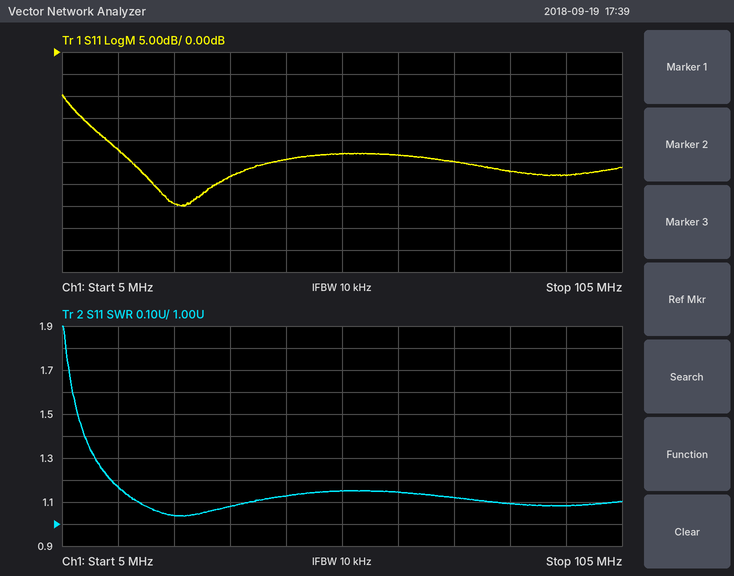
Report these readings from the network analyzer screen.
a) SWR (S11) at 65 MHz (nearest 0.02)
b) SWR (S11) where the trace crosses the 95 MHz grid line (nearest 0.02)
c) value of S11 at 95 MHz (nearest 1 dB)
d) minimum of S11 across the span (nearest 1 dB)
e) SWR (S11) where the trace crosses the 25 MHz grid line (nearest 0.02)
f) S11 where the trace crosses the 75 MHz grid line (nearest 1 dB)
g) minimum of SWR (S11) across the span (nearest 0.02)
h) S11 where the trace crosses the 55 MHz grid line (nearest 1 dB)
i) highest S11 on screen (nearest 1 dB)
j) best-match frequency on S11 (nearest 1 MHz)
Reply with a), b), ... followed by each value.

a) 1.14
b) 1.08
c) -28 dB
d) -35 dB
e) 1.04
f) -25 dB
g) 1.04
h) -23 dB
i) -10 dB
j) 27 MHz
